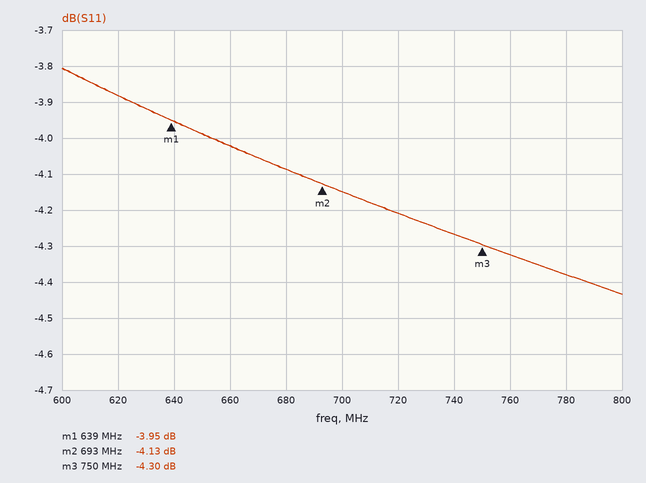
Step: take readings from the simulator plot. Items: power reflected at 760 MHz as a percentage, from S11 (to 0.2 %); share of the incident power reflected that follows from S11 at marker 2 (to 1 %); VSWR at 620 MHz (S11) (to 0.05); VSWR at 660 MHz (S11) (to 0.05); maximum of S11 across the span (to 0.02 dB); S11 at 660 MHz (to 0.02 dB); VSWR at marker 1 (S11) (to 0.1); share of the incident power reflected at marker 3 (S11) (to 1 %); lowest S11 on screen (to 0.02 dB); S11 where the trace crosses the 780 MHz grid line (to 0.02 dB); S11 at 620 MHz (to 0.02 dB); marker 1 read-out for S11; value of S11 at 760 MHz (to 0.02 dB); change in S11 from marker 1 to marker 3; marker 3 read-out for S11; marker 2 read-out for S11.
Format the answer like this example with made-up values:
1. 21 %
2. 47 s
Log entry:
1. 37.0 %
2. 39 %
3. 4.55
4. 4.40
5. -3.80 dB
6. -4.02 dB
7. 4.5
8. 37 %
9. -4.44 dB
10. -4.38 dB
11. -3.88 dB
12. -3.95 dB
13. -4.32 dB
14. -0.35 dB
15. -4.30 dB
16. -4.13 dB
